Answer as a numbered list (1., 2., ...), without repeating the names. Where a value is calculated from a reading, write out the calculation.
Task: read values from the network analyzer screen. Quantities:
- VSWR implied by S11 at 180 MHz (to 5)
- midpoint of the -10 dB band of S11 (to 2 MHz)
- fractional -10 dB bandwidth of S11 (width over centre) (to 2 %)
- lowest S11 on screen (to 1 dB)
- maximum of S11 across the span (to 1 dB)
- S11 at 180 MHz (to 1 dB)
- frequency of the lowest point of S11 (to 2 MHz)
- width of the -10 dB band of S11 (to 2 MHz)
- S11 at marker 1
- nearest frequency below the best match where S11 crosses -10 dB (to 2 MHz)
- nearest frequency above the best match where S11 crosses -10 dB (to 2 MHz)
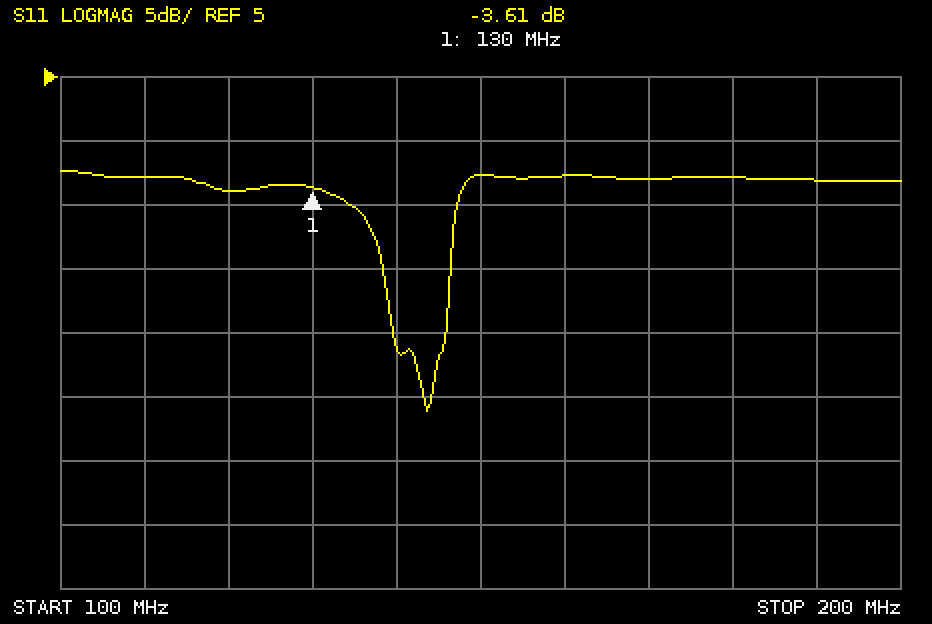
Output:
1. |Γ| = 10^(-3/20) = 0.7079; VSWR = (1 + 0.7079)/(1 − 0.7079) ≈ 5.85, so 5 to the nearest 5
2. 142 MHz
3. 8 MHz / 142 MHz ≈ 6 %
4. -21 dB
5. -2 dB
6. -3 dB
7. 144 MHz
8. 146 MHz − 138 MHz = 8 MHz
9. -3.61 dB
10. 138 MHz
11. 146 MHz
